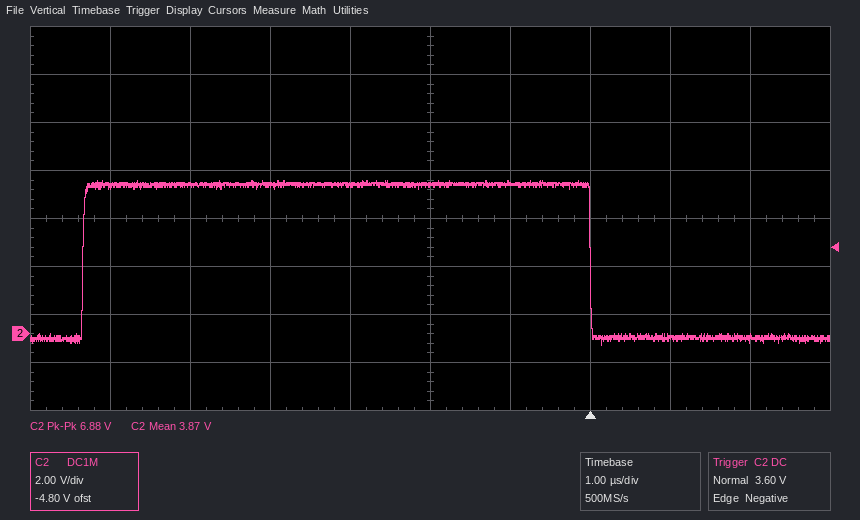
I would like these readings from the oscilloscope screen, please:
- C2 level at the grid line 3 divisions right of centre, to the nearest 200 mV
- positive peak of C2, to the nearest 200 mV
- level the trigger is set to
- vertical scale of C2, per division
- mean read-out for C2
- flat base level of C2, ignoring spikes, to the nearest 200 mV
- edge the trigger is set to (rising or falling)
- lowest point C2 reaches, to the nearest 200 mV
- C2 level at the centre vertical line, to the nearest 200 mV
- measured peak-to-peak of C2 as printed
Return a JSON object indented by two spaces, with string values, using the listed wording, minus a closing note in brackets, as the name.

{
  "C2 level at the grid line 3 divisions right of centre, to the nearest 200 mV": "-200 mV",
  "positive peak of C2, to the nearest 200 mV": "6.4 V",
  "level the trigger is set to": "3.60 V",
  "vertical scale of C2, per division": "2 V",
  "mean read-out for C2": "3.87 V",
  "flat base level of C2, ignoring spikes, to the nearest 200 mV": "-200 mV",
  "edge the trigger is set to": "falling",
  "lowest point C2 reaches, to the nearest 200 mV": "-400 mV",
  "C2 level at the centre vertical line, to the nearest 200 mV": "6.2 V",
  "measured peak-to-peak of C2 as printed": "6.88 V"
}
